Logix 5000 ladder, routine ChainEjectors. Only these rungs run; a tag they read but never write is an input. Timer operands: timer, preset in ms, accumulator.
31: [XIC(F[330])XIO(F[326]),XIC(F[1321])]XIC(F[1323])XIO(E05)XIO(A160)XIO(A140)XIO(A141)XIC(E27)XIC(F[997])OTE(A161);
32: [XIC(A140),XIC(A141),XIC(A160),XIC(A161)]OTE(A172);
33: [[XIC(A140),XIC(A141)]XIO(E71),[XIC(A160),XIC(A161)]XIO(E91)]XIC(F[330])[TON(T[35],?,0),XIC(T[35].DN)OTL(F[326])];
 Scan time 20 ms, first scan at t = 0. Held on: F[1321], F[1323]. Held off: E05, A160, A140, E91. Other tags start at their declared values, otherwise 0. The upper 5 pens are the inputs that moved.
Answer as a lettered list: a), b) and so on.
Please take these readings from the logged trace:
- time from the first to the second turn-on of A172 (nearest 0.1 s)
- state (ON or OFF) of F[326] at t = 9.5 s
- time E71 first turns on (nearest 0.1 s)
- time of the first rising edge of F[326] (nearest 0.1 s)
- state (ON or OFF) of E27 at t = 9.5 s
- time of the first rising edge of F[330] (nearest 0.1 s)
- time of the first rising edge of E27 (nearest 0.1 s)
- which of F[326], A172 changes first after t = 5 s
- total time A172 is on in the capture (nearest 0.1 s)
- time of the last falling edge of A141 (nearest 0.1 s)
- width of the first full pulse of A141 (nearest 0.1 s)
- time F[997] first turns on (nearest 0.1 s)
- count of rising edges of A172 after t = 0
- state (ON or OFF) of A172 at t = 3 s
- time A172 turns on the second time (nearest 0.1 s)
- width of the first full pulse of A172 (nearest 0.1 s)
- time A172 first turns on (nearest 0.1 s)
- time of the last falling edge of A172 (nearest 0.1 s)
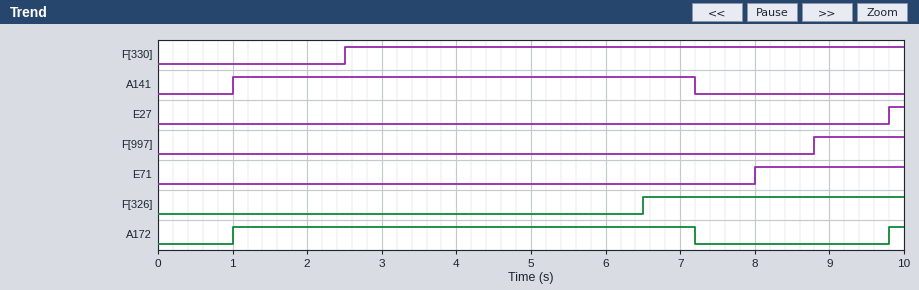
a) 8.8 s
b) ON
c) 8.0 s
d) 6.5 s
e) OFF
f) 2.5 s
g) 9.8 s
h) F[326]
i) 6.4 s
j) 7.2 s
k) 6.2 s
l) 8.8 s
m) 2
n) ON
o) 9.8 s
p) 6.2 s
q) 1.0 s
r) 7.2 s
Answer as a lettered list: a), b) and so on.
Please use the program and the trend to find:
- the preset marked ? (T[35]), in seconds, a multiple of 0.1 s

a) 4.0 s
